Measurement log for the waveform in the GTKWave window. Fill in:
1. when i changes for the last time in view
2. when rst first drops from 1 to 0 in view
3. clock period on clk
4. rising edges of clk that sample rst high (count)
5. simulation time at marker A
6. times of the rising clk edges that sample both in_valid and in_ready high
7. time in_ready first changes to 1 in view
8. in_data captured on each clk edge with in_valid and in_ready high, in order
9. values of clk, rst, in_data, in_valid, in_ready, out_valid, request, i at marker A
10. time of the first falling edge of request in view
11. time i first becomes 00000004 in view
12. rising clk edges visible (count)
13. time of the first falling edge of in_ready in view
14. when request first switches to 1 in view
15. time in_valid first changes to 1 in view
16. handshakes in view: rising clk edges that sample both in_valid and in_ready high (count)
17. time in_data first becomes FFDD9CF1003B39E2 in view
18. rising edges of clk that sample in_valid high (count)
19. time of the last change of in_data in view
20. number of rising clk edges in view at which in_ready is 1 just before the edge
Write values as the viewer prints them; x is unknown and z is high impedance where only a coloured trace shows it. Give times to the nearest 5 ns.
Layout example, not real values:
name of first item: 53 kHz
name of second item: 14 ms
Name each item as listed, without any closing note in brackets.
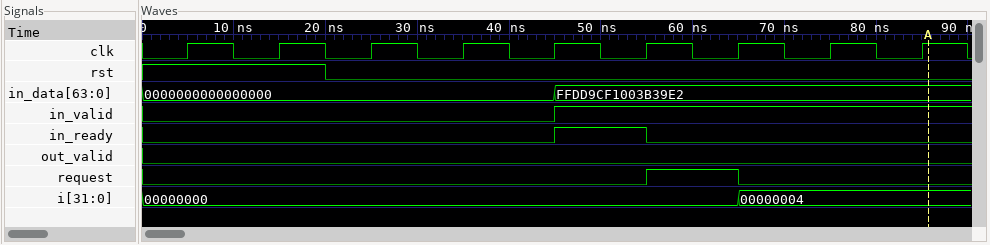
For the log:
when i changes for the last time in view: 65 ns
when rst first drops from 1 to 0 in view: 20 ns
clock period on clk: 10 ns
rising edges of clk that sample rst high: 2
simulation time at marker A: 85 ns
times of the rising clk edges that sample both in_valid and in_ready high: 55 ns
time in_ready first changes to 1 in view: 45 ns
in_data captured on each clk edge with in_valid and in_ready high, in order: FFDD9CF1003B39E2
values of clk, rst, in_data, in_valid, in_ready, out_valid, request, i at marker A: clk=1, rst=0, in_data=FFDD9CF1003B39E2, in_valid=1, in_ready=0, out_valid=0, request=0, i=00000004
time of the first falling edge of request in view: 65 ns
time i first becomes 00000004 in view: 65 ns
rising clk edges visible: 9
time of the first falling edge of in_ready in view: 55 ns
when request first switches to 1 in view: 55 ns
time in_valid first changes to 1 in view: 45 ns
handshakes in view: rising clk edges that sample both in_valid and in_ready high: 1
time in_data first becomes FFDD9CF1003B39E2 in view: 45 ns
rising edges of clk that sample in_valid high: 4
time of the last change of in_data in view: 45 ns
number of rising clk edges in view at which in_ready is 1 just before the edge: 1
